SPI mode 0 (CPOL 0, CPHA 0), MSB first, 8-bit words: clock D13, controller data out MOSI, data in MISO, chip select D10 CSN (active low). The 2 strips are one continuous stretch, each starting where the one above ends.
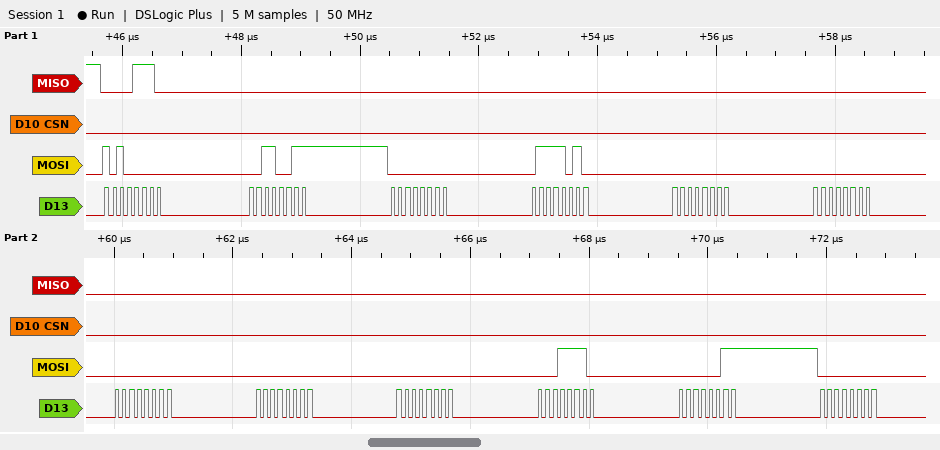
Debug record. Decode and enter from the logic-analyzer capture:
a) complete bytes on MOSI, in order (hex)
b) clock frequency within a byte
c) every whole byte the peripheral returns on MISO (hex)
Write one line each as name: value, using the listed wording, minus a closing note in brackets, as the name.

complete bytes on MOSI, in order: 0xA0 0x33 0x00 0x7A 0x00 0x00 0x00 0x00 0x00 0x1E 0x03 0x00
clock frequency within a byte: 8 MHz
every whole byte the peripheral returns on MISO: 0x0E 0x00 0x00 0x00 0x00 0x00 0x00 0x00 0x00 0x00 0x00 0x00
